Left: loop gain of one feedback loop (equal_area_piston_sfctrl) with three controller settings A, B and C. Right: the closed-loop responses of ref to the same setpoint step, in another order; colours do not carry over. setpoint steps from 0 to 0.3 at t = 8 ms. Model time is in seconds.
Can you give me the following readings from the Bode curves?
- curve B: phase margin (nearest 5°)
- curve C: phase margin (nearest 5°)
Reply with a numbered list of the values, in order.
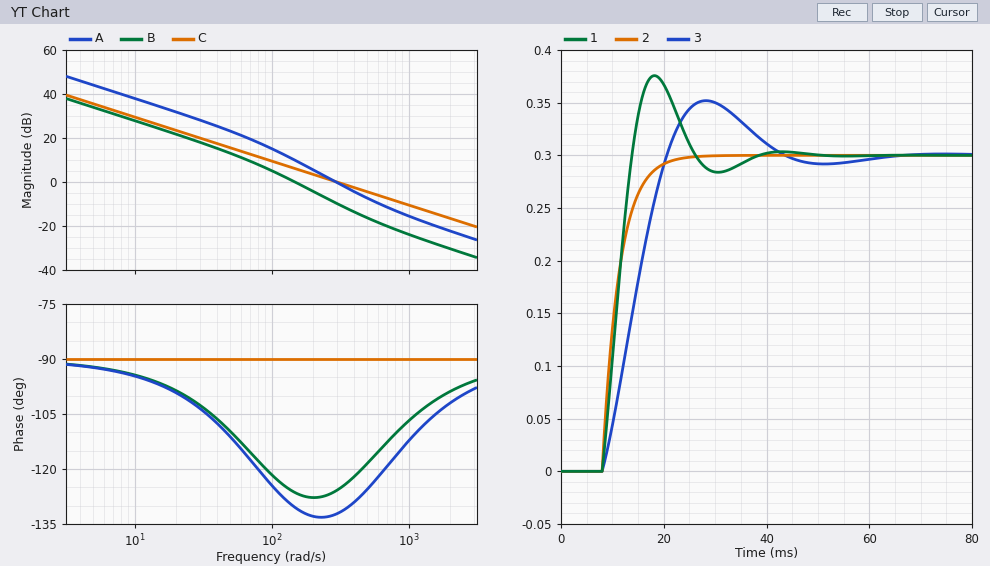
1. 55°
2. 90°
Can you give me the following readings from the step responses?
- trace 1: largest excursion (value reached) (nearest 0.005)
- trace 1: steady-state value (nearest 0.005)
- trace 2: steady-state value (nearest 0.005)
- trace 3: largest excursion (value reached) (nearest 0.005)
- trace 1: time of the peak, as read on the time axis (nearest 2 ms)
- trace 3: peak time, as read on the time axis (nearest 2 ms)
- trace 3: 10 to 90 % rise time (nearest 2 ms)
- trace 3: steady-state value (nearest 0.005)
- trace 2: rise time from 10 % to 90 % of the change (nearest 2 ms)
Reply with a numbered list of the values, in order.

1. 0.375
2. 0.300
3. 0.300
4. 0.350
5. 18 ms
6. 28 ms
7. 10 ms
8. 0.300
9. 8 ms
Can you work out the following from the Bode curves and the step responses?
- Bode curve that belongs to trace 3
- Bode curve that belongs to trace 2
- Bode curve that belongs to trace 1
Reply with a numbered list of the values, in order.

1. B
2. C
3. A
